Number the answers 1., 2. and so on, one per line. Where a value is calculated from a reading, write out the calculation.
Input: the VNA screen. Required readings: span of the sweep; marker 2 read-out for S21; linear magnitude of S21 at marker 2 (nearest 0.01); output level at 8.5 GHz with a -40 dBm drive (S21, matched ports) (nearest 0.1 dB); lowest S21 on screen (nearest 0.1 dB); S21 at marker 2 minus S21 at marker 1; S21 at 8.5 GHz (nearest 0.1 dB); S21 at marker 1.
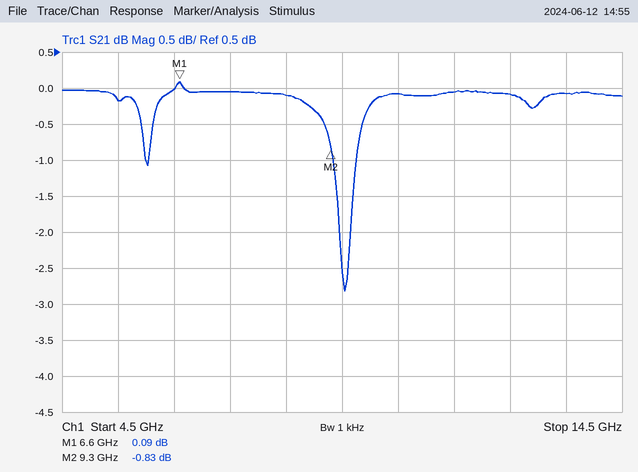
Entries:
1. 10 GHz
2. -0.83 dB
3. 10^(-0.83/20) ≈ 0.91
4. -40 dBm + (-0.1 dB) = -40.1 dBm
5. -2.8 dB
6. -0.83 − (0.09) = -0.92 dB
7. -0.1 dB
8. 0.09 dB
